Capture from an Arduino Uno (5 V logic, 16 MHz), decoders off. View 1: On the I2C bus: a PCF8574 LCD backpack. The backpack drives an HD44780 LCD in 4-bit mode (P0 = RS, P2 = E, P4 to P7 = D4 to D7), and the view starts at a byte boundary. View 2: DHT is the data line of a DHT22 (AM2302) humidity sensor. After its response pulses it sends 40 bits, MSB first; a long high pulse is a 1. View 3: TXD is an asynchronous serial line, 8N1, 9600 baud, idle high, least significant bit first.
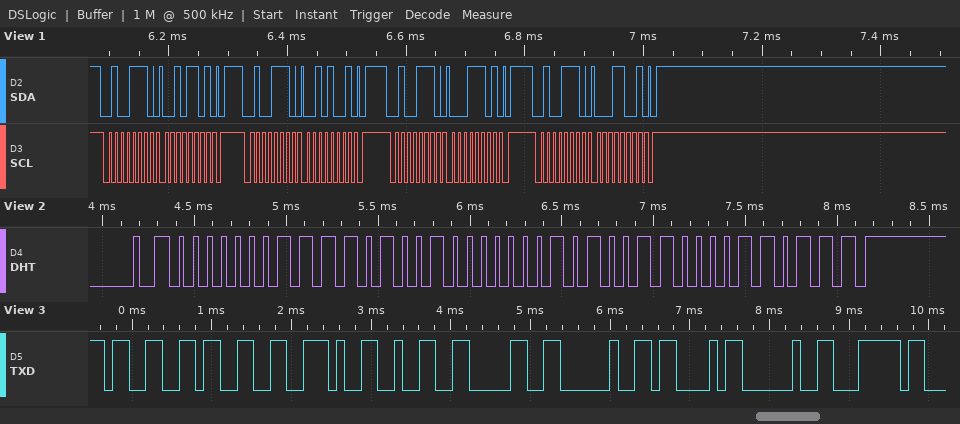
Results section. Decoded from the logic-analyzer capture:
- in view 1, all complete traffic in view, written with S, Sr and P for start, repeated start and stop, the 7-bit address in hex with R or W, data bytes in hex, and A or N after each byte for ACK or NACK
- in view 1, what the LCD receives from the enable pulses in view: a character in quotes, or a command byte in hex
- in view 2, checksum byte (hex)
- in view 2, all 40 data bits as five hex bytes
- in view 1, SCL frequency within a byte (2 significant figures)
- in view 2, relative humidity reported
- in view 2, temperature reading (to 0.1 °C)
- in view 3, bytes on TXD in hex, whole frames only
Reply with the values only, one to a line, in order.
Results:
S 27W A 2D A P S 27W A 29 A P S 27W A 1D A P S 27W A 19 A P
'!'
0x37
01 E9 01 4C 37
100 kHz
48.9 %
33.2 °C
33 33 2E 32 30 20 43 20 7C
